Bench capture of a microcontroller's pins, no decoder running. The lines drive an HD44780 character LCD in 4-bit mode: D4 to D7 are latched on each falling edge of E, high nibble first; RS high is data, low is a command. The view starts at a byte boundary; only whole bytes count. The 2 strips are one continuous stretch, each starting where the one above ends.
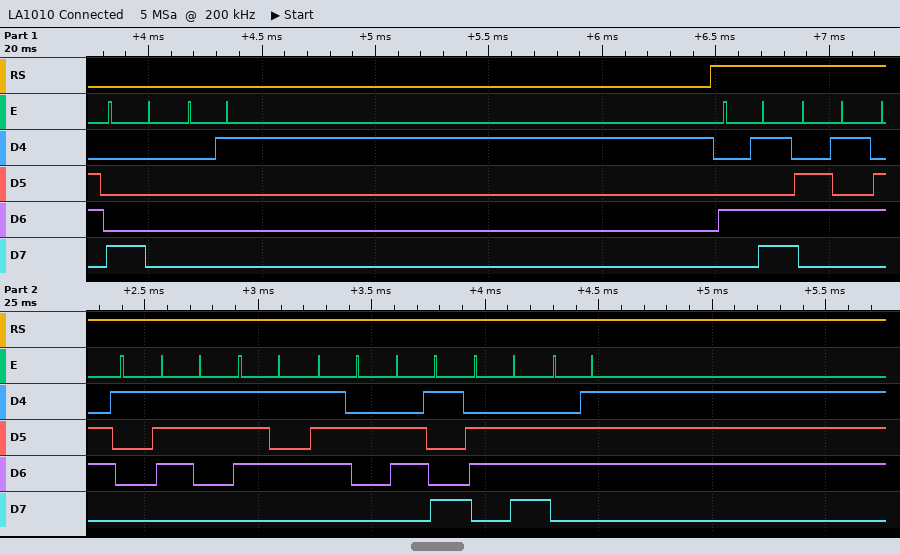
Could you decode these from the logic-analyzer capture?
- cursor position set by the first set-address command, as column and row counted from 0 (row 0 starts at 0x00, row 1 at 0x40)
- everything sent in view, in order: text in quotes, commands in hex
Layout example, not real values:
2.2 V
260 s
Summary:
column 0, row 0
0x80 0x01 "Measuring"
